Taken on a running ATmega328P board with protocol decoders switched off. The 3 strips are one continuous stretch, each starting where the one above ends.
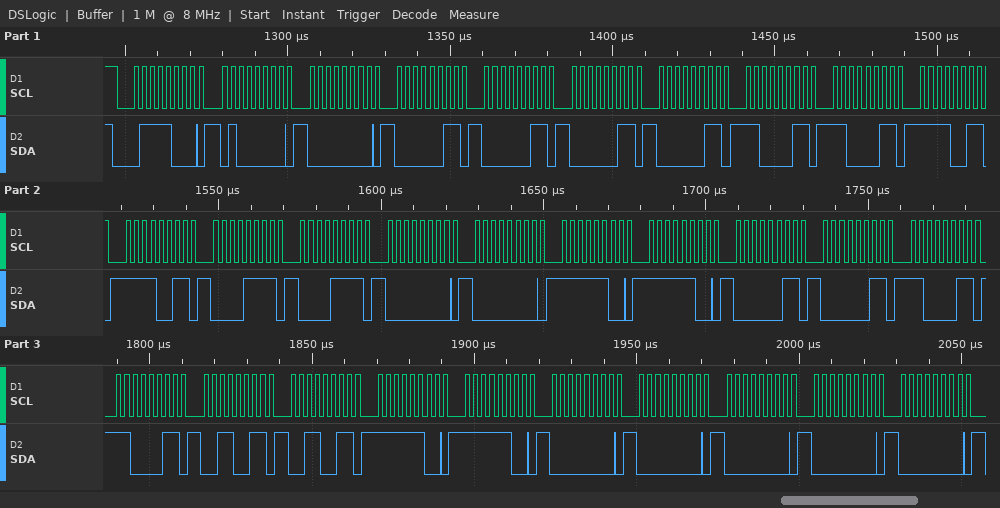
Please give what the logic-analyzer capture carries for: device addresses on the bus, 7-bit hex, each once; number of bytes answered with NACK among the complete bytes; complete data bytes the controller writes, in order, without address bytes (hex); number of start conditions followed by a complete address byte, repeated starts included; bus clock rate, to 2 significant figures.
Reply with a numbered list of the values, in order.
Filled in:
1. 0x3C
2. 0
3. 40 00 03 03 03 03 C3 C3 F3 F3 0F 0F 00 00 FC FC 03 03 C3 C3 33 33 FC FC 00 00 00 00 00
4. 1
5. 400 kHz
